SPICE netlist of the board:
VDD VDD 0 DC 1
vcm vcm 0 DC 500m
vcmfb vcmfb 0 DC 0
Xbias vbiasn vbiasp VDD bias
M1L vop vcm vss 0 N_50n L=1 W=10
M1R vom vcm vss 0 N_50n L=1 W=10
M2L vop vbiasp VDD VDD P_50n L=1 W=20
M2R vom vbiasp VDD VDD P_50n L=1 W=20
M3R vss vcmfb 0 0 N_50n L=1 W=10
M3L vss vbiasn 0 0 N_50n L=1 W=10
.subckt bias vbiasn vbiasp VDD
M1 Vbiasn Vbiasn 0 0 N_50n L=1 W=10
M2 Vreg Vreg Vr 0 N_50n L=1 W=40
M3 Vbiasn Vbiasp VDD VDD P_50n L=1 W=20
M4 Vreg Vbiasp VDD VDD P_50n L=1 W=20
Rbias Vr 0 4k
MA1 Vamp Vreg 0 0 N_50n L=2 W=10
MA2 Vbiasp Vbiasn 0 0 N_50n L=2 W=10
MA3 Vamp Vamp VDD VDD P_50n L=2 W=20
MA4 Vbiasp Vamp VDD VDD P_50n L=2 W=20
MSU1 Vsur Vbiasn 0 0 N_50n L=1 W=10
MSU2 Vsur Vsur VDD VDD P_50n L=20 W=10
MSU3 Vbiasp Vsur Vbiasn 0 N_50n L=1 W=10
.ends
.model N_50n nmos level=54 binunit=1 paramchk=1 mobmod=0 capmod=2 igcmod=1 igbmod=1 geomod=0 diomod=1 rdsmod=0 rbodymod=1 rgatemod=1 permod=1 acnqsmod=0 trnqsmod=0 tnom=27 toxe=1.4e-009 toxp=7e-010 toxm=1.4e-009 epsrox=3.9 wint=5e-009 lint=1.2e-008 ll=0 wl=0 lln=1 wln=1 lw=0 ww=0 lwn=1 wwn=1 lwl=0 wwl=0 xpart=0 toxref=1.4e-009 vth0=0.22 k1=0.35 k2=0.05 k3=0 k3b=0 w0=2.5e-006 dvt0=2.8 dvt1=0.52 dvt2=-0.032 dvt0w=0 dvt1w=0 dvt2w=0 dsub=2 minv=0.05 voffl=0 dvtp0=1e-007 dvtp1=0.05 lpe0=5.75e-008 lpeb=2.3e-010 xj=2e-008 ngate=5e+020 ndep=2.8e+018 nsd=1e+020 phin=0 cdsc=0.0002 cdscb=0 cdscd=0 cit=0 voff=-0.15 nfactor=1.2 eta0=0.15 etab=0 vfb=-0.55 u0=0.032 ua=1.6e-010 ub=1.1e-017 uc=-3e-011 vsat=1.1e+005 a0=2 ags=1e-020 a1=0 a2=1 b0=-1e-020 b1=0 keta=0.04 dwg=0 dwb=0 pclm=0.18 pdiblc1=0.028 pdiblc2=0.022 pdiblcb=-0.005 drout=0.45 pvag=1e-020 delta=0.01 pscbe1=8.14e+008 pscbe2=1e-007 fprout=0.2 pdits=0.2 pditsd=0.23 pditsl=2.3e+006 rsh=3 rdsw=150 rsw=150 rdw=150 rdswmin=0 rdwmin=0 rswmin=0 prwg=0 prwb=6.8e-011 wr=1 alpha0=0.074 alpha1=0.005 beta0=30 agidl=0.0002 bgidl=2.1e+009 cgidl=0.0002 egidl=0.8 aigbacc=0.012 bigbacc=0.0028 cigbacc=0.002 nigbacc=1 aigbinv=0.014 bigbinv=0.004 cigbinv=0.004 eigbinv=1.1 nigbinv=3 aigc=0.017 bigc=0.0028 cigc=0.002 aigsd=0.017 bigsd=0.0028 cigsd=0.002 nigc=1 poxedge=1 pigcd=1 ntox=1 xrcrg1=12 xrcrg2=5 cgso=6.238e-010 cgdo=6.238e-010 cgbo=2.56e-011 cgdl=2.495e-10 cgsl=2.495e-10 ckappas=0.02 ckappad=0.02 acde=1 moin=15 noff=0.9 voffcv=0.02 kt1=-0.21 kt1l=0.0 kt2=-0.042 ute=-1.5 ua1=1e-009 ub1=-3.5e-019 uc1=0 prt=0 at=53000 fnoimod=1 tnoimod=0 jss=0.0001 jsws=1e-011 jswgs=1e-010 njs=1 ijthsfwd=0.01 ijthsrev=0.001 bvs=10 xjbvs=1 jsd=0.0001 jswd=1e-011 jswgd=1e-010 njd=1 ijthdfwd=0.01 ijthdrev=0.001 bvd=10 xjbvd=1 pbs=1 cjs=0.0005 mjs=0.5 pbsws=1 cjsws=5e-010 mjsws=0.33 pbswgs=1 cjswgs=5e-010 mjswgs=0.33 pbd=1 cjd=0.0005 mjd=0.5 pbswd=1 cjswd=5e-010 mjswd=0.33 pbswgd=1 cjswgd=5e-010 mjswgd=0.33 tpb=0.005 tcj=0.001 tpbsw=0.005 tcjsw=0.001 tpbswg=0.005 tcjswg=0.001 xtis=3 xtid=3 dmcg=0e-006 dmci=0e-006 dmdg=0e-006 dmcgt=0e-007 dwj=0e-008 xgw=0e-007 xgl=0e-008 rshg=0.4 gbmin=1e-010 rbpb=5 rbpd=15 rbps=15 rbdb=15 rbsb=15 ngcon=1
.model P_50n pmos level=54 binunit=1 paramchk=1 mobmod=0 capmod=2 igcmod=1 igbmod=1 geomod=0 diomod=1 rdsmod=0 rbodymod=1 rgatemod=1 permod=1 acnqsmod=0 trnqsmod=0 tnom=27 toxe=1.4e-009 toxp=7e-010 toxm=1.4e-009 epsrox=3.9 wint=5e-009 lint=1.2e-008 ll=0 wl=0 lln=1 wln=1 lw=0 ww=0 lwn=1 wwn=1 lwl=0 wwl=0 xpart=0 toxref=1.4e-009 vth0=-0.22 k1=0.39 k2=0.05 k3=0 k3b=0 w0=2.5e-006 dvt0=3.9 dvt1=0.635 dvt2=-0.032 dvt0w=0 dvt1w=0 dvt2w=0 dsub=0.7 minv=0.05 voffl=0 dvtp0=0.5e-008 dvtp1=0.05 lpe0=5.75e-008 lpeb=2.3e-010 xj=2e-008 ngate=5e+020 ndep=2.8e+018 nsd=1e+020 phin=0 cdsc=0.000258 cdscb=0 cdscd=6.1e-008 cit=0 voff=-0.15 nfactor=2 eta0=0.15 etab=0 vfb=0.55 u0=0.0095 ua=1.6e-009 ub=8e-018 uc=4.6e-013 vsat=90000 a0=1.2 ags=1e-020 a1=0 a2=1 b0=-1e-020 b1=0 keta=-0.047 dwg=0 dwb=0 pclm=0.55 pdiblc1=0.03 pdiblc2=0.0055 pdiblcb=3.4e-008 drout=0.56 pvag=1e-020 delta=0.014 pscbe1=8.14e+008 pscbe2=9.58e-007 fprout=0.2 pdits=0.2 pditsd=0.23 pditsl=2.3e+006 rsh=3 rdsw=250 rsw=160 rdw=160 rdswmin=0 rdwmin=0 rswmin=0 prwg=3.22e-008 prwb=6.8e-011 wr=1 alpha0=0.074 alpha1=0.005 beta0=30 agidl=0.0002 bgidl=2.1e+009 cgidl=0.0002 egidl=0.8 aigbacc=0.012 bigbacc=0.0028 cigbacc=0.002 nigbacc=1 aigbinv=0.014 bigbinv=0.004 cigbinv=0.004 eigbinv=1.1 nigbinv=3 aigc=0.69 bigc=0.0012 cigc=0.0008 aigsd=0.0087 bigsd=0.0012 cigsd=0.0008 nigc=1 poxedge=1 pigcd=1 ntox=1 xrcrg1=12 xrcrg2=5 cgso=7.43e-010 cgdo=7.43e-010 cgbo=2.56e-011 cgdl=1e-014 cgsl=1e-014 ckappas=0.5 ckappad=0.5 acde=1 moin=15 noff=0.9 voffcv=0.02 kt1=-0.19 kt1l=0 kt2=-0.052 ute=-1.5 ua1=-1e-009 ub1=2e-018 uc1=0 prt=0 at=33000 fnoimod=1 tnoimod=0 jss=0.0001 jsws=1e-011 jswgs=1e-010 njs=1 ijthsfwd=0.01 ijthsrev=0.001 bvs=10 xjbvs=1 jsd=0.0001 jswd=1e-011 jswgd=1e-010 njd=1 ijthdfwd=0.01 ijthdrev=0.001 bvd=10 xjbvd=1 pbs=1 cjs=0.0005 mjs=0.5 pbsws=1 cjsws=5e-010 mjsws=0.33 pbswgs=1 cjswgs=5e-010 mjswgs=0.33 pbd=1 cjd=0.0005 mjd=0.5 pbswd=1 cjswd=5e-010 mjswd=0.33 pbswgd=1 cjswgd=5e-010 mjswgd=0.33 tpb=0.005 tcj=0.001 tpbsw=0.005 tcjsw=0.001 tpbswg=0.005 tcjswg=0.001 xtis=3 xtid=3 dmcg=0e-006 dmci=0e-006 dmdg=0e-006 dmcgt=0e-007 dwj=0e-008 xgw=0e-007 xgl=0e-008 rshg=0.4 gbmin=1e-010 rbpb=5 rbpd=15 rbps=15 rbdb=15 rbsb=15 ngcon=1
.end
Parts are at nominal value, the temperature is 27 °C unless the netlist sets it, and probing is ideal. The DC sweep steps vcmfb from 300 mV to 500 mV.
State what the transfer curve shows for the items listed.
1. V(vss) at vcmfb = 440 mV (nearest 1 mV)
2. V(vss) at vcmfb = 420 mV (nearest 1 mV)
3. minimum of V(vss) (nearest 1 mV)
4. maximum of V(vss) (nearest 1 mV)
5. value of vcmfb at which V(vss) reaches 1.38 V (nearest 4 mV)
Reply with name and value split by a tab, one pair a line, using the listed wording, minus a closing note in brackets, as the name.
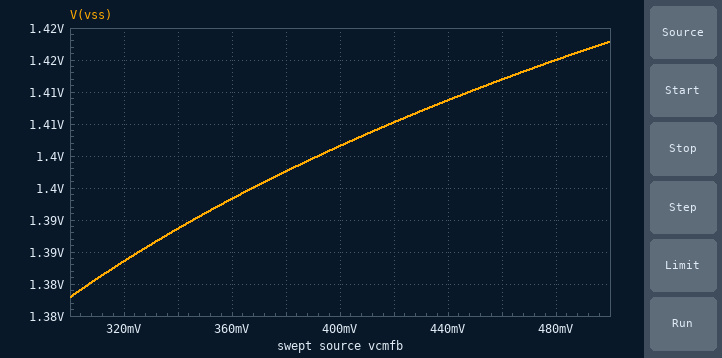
V(vss) at vcmfb = 440 mV	1.409 V
V(vss) at vcmfb = 420 mV	1.405 V
minimum of V(vss)	1.378 V
maximum of V(vss)	1.418 V
value of vcmfb at which V(vss) reaches 1.38 V	308 mV
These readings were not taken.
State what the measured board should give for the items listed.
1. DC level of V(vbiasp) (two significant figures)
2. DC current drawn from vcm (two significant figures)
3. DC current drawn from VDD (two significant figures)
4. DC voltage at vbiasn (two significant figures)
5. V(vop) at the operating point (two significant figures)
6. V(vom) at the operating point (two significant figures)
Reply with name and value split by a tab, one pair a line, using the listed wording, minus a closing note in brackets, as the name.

DC level of V(vbiasp)	960 mV
DC current drawn from vcm	99 mA
DC current drawn from VDD	210 mA
DC voltage at vbiasn	82 mV
V(vop) at the operating point	870 mV
V(vom) at the operating point	870 mV
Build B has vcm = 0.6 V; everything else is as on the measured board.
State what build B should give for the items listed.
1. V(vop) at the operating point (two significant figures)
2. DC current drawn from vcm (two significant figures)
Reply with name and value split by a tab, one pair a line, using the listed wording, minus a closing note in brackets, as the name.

V(vop) at the operating point	890 mV
DC current drawn from vcm	130 mA
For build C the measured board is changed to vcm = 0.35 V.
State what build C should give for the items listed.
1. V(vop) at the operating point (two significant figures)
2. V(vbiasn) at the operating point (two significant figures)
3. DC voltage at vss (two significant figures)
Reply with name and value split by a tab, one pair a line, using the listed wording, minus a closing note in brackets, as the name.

V(vop) at the operating point	840 mV
V(vbiasn) at the operating point	82 mV
DC voltage at vss	990 mV
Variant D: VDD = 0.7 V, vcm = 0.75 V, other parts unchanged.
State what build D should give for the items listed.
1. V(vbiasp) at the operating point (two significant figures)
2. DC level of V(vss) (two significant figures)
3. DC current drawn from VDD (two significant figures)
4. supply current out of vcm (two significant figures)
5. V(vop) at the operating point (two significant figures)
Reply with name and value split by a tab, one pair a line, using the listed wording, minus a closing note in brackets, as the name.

V(vbiasp) at the operating point	720 mV
DC level of V(vss)	900 mV
DC current drawn from VDD	110 mA
supply current out of vcm	170 mA
V(vop) at the operating point	640 mV
